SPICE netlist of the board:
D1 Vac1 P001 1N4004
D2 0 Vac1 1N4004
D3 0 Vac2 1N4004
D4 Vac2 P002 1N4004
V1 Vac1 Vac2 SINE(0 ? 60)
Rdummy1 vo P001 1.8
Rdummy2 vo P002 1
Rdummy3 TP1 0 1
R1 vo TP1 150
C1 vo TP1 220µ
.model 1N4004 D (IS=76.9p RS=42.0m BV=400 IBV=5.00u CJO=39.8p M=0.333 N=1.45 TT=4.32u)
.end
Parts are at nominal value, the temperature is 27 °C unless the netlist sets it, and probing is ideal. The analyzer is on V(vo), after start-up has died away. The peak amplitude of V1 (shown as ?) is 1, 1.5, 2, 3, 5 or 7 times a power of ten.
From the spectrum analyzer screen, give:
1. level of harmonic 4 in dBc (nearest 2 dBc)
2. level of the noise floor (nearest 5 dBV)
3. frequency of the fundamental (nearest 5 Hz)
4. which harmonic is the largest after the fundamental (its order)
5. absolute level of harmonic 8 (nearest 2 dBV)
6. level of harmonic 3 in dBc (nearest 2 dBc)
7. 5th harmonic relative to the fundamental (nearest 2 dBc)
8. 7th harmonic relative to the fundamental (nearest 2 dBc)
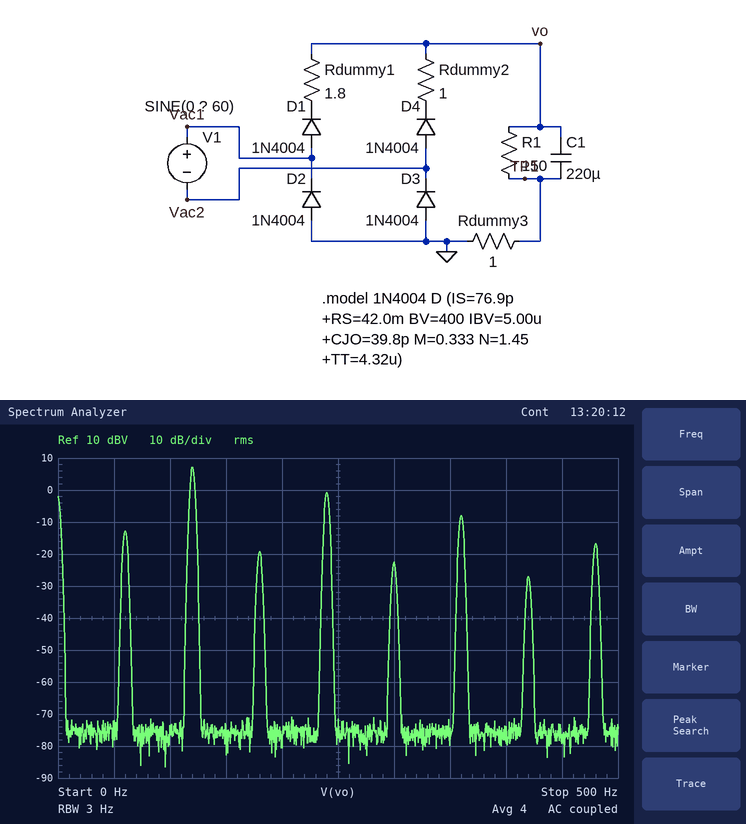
12 dBc
-75 dBV
60 Hz
2
-16 dBV
-6 dBc
-10 dBc
-14 dBc
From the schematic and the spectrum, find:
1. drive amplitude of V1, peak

50 V
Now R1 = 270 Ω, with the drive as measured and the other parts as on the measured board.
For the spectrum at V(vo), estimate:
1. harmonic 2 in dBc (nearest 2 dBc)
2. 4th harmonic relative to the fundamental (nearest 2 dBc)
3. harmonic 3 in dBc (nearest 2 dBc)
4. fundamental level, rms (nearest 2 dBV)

18 dBc
10 dBc
-8 dBc
-16 dBV
